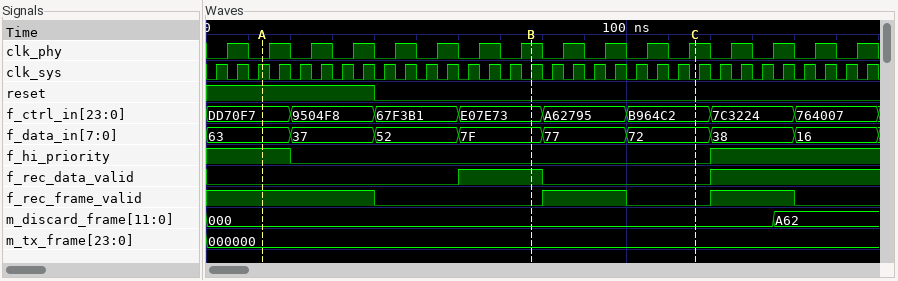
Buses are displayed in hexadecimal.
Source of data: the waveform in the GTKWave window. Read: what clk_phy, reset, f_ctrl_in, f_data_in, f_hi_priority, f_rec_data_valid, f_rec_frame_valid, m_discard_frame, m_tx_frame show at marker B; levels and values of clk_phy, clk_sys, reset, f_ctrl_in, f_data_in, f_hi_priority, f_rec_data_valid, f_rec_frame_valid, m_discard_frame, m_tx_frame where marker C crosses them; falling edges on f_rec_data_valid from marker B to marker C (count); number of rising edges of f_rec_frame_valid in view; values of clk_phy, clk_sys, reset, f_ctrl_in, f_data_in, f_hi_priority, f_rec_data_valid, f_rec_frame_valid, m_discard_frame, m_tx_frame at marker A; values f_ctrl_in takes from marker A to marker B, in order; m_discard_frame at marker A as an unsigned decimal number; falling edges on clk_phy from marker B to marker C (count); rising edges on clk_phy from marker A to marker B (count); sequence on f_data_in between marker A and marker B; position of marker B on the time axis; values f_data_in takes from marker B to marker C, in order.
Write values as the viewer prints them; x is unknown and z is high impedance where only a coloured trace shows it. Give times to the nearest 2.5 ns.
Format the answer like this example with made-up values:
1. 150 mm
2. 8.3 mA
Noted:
1. clk_phy=1, reset=0, f_ctrl_in=E07E73, f_data_in=7F, f_hi_priority=0, f_rec_data_valid=1, f_rec_frame_valid=0, m_discard_frame=000, m_tx_frame=000000
2. clk_phy=1, clk_sys=0, reset=0, f_ctrl_in=B964C2, f_data_in=72, f_hi_priority=0, f_rec_data_valid=0, f_rec_frame_valid=0, m_discard_frame=000, m_tx_frame=000000
3. 1
4. 2
5. clk_phy=0, clk_sys=1, reset=1, f_ctrl_in=DD70F7, f_data_in=63, f_hi_priority=1, f_rec_data_valid=0, f_rec_frame_valid=1, m_discard_frame=000, m_tx_frame=000000
6. DD70F7, 9504F8, 67F3B1, E07E73
7. 0
8. 4
9. 7
10. 63, 37, 52, 7F
11. 77.5 ns
12. 7F, 77, 72
